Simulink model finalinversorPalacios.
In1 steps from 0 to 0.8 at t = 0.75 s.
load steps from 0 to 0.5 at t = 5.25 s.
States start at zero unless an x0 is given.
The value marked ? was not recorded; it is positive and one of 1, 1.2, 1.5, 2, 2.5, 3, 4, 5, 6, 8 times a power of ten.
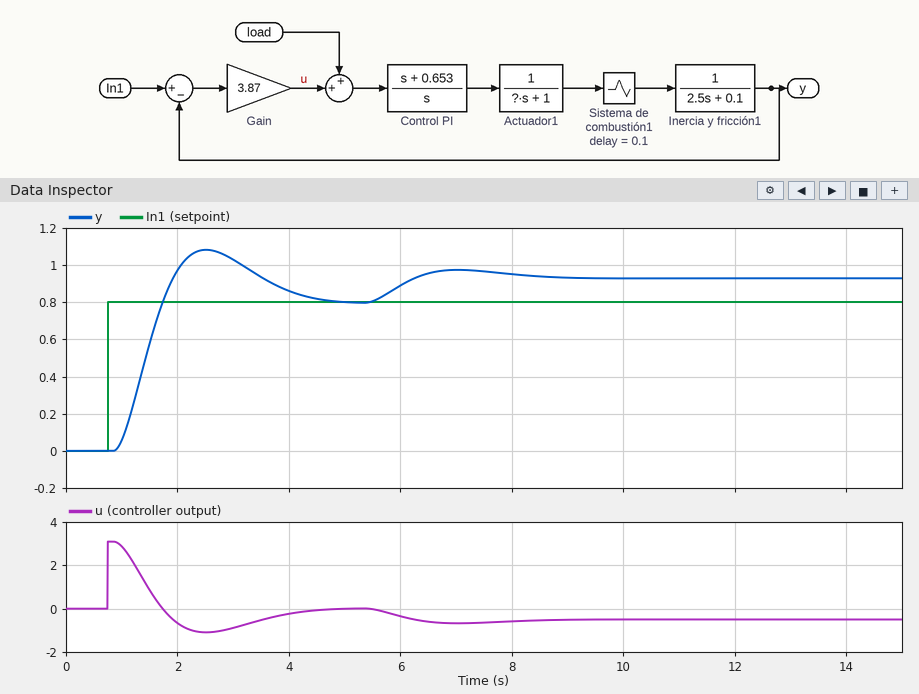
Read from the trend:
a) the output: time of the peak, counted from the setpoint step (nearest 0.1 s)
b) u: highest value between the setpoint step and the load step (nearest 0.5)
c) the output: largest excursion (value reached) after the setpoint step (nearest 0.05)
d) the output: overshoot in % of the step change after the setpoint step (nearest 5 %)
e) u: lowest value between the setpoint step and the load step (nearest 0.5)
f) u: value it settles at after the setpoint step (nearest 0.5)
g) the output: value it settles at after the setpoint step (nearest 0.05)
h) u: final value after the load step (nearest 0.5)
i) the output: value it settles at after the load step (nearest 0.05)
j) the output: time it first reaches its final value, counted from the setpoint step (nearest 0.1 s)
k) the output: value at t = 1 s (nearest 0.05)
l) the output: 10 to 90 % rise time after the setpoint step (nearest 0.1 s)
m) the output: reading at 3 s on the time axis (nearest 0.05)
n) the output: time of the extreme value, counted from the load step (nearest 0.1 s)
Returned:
1.8 s
3.0
1.10
35 %
-1.0
0.0
0.80
-0.5
0.95
1.0 s
0.05
0.6 s
1.05
1.8 s
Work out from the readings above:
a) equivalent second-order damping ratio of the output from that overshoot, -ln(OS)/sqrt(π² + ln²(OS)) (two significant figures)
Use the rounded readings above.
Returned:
0.32
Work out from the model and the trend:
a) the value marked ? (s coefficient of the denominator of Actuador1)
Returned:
0.2
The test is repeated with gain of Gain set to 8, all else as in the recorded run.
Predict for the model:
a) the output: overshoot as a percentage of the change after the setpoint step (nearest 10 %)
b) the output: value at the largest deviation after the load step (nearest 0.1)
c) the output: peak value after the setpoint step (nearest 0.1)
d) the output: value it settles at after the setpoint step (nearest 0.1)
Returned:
50 %
0.9
1.2
0.8
